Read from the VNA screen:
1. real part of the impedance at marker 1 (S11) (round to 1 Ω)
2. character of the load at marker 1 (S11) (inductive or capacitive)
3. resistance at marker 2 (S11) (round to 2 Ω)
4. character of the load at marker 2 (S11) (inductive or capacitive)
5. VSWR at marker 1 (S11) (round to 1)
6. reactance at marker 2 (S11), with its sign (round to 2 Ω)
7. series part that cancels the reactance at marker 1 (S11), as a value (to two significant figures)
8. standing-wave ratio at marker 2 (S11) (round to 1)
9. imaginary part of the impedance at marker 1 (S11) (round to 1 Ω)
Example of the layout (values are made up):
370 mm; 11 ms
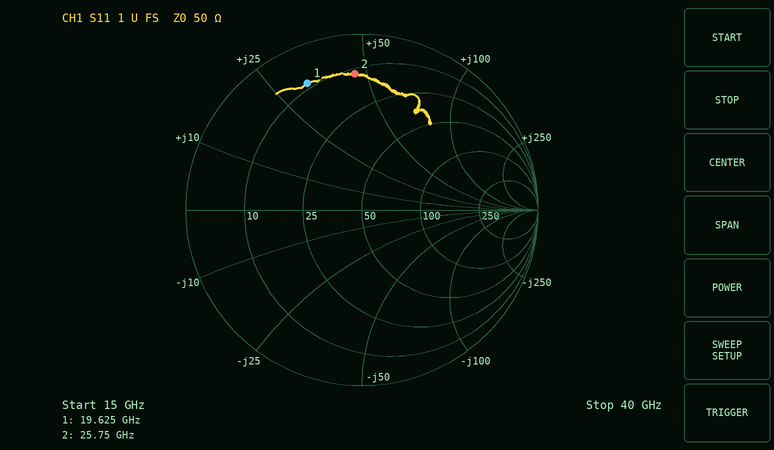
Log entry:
9 Ω; inductive; 12 Ω; inductive; 8; +46 Ω; 250 fF; 8; +32 Ω
